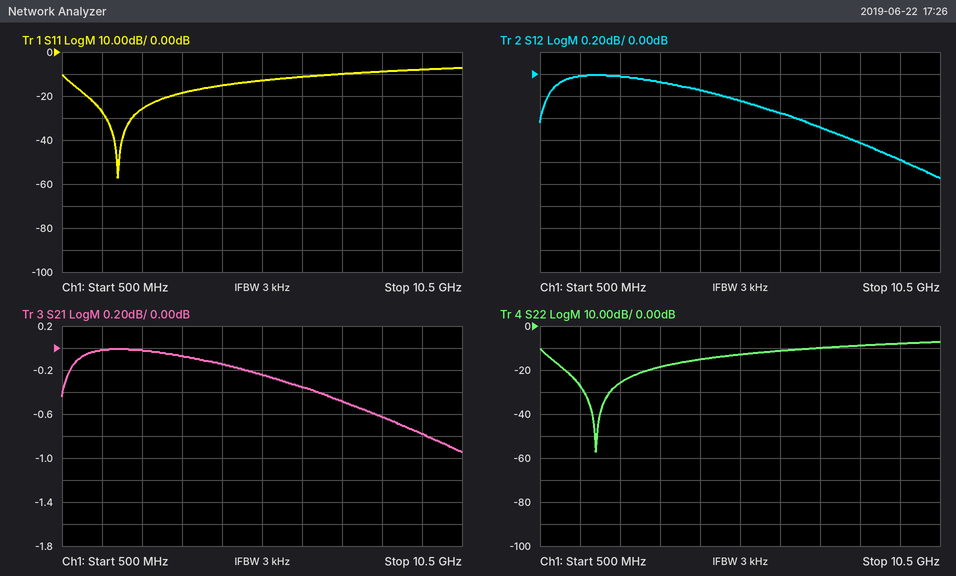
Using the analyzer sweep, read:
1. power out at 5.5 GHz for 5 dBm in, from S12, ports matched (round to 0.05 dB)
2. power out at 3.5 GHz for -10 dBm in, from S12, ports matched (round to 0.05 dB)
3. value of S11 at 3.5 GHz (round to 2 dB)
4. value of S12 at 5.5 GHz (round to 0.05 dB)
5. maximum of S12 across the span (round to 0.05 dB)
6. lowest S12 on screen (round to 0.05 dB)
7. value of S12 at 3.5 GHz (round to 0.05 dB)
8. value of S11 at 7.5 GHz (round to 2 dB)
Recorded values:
4.75 dBm
-10.05 dBm
-18 dB
-0.25 dB
0.00 dB
-0.95 dB
-0.05 dB
-10 dB
